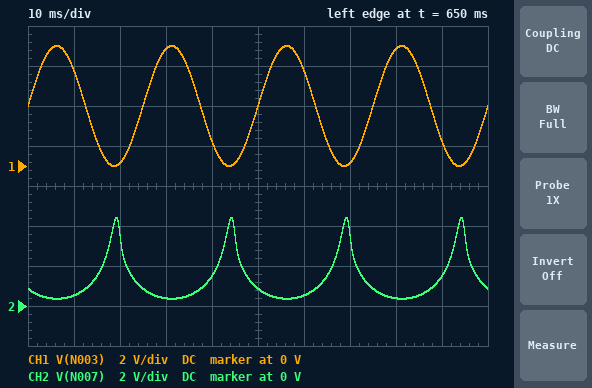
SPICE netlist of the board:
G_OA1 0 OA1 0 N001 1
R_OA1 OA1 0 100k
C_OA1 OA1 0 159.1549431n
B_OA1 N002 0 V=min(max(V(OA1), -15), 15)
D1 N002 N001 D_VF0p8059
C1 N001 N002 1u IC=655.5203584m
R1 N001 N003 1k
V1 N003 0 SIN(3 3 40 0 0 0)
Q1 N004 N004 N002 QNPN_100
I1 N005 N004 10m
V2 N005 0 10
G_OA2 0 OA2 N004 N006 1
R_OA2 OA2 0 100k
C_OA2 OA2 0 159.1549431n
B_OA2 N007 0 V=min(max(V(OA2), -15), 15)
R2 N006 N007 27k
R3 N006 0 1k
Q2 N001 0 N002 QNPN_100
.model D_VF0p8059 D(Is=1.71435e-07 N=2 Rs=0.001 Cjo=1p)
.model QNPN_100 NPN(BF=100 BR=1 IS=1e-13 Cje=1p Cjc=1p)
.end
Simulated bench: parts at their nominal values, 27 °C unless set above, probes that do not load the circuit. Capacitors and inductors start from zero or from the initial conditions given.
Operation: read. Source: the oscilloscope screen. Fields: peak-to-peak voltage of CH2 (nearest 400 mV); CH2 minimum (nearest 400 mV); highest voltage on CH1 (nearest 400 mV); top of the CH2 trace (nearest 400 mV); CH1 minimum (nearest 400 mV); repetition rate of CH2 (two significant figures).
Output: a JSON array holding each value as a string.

["4.0 V", "400 mV", "6.0 V", "4.4 V", "0 V", "40 Hz"]
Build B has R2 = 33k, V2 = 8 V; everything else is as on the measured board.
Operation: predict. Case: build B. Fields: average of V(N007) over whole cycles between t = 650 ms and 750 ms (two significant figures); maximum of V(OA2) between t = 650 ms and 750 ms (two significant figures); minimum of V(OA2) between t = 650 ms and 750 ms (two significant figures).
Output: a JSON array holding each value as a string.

["1.6 V", "5.4 V", "440 mV"]
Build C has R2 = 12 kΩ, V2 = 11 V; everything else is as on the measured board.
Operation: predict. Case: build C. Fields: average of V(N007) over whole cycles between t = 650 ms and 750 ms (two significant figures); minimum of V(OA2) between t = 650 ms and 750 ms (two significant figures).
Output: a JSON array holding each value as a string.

["610 mV", "170 mV"]
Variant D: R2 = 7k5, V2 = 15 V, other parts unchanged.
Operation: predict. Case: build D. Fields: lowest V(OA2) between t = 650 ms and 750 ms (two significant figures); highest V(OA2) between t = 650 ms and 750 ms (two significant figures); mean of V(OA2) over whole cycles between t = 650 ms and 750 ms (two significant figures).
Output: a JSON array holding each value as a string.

["110 mV", "1.3 V", "400 mV"]
